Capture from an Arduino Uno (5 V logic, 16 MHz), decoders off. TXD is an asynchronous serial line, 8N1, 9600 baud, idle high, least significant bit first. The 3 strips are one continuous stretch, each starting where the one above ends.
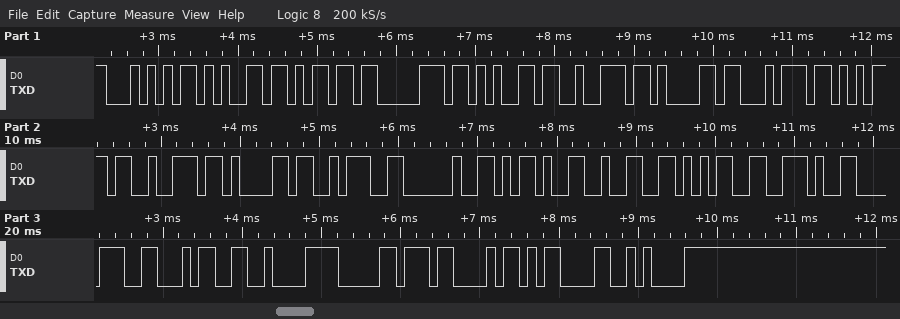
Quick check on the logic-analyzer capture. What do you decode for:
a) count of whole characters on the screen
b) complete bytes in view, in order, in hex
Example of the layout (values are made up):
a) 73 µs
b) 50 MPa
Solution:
a) 24
b) 54 65 6D 70 65 72 61 74 75 72 61 3A 20 2D 32 35 2E 38 34 C2 B0 43 0D 0A
